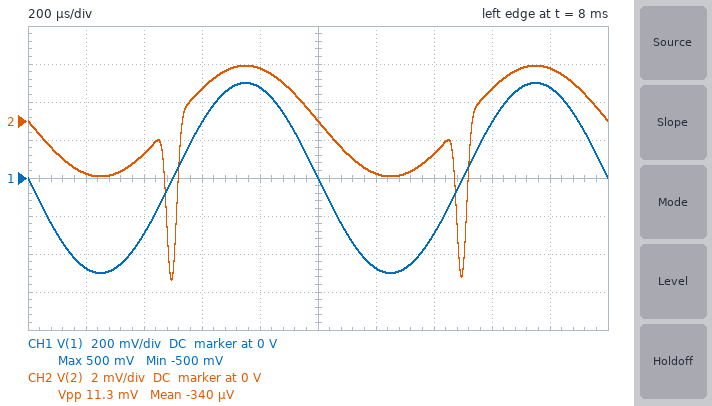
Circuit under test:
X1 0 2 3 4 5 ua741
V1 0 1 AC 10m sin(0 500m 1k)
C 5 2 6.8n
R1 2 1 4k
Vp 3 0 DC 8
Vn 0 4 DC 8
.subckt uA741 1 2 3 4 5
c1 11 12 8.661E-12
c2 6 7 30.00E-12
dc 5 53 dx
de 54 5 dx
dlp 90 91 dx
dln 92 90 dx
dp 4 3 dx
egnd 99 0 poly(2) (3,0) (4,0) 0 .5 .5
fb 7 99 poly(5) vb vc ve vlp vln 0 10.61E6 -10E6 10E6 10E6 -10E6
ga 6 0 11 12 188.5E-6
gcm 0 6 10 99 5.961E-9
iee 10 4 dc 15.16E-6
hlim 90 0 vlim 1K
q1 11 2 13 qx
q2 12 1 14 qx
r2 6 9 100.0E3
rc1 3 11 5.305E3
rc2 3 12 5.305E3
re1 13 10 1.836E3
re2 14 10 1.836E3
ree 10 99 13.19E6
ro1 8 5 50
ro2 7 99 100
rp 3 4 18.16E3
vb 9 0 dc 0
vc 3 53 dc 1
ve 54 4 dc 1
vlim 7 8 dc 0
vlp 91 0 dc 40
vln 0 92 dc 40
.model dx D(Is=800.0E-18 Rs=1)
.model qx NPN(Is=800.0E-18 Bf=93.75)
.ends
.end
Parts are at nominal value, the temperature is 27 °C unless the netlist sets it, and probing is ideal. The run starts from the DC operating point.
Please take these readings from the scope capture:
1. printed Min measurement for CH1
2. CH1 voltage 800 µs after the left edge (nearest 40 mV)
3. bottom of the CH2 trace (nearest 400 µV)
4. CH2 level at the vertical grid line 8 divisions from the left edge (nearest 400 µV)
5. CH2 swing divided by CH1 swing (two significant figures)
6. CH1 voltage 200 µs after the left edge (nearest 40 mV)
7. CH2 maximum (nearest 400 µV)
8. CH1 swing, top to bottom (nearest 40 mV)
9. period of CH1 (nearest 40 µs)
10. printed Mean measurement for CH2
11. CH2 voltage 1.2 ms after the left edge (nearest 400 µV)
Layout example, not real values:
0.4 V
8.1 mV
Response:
-500 mV
480 mV
-8.4 mV
1.6 mV
0.011
-480 mV
2.8 mV
1.00 V
1.00 ms
-340 µV
-2.8 mV
